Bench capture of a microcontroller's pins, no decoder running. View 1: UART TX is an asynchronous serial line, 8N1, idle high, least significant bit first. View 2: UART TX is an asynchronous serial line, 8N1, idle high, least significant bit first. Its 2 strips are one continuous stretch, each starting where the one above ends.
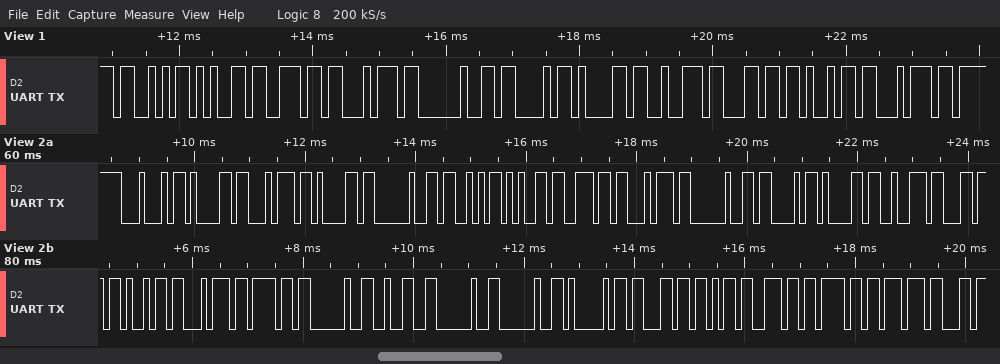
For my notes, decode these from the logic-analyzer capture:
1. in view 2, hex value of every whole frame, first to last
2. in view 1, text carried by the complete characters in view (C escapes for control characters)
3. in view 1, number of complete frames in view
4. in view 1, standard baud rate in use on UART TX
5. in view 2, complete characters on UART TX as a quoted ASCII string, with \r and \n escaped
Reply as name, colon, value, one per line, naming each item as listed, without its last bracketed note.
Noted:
in view 2, hex value of every whole frame, first to last: 44 61 74 61 20 53 65 6E 74 20 43 61 72 6C 69 74 6F 20 32 20 20 41 63 6B 6E 6F 77
in view 1, text carried by the complete characters in view: "Sent Carlit"
in view 1, number of complete frames in view: 11
in view 1, standard baud rate in use on UART TX: 9600 baud
in view 2, complete characters on UART TX as a quoted ASCII string, with \r and \n escaped: "Data Sent Carlito 2  Acknow"
